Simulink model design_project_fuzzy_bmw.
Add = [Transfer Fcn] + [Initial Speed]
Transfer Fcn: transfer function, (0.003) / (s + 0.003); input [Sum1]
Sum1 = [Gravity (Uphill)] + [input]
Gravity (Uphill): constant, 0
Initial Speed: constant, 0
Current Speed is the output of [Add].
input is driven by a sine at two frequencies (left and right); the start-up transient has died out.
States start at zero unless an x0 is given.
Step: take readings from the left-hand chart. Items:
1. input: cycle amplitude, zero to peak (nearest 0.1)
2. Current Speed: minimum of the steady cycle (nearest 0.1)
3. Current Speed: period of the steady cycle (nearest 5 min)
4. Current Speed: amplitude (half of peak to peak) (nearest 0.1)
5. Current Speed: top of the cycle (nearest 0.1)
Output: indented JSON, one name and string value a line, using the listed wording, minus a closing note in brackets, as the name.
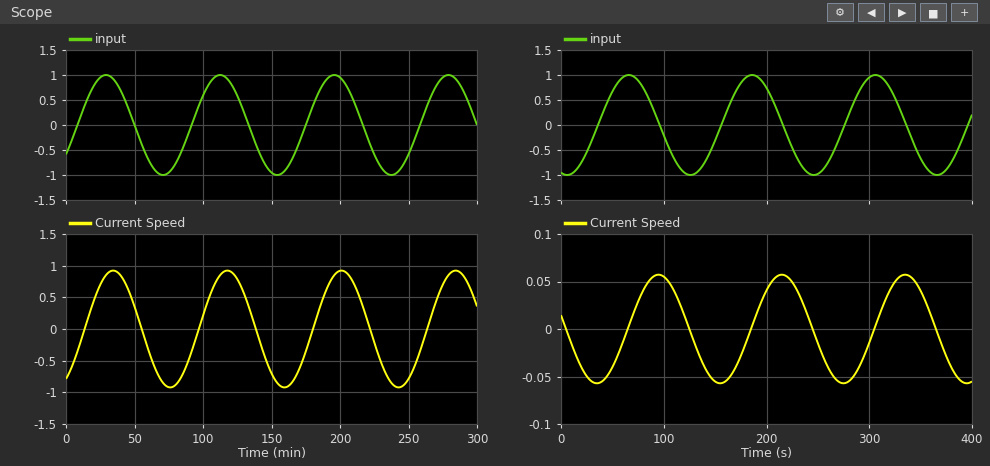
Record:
{
  "input: cycle amplitude, zero to peak": "1.0",
  "Current Speed: minimum of the steady cycle": "-0.9",
  "Current Speed: period of the steady cycle": "85 min",
  "Current Speed: amplitude (half of peak to peak)": "0.9",
  "Current Speed: top of the cycle": "0.9"
}
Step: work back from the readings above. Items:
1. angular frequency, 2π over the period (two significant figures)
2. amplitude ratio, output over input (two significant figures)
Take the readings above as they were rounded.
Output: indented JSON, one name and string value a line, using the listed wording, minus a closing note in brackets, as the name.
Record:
{
  "angular frequency, 2π over the period": "0.074 rad/min",
  "amplitude ratio, output over input": "0.90"
}
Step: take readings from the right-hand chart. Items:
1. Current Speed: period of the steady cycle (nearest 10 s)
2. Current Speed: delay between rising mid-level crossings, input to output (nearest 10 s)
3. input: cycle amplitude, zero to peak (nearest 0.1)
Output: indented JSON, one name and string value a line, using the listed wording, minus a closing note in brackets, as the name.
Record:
{
  "Current Speed: period of the steady cycle": "120 s",
  "Current Speed: delay between rising mid-level crossings, input to output": "30 s",
  "input: cycle amplitude, zero to peak": "1.0"
}
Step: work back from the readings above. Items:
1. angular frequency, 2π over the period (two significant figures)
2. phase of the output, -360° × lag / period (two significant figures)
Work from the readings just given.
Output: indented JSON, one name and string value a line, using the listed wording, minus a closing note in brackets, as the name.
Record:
{
  "angular frequency, 2π over the period": "0.052 rad/s",
  "phase of the output, -360° × lag / period": "-90°"
}
